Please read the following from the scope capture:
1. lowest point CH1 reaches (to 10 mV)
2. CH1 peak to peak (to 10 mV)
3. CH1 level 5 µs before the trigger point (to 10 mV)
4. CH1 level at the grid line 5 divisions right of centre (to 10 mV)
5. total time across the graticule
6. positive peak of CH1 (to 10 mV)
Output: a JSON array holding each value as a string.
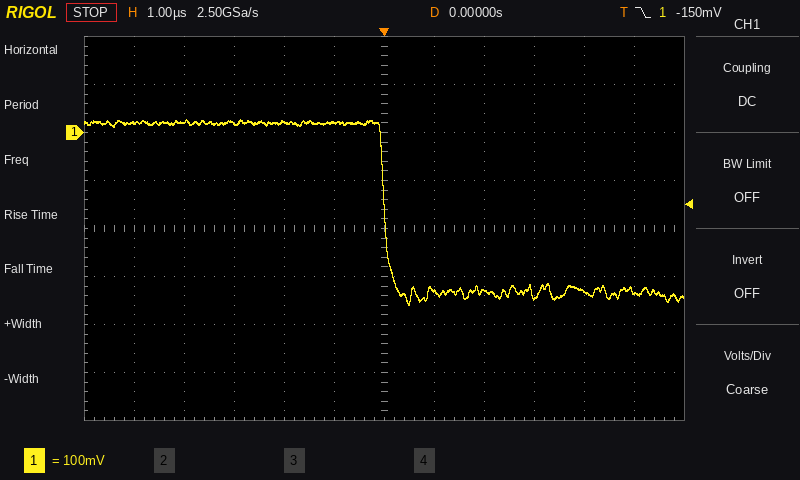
["-360 mV", "390 mV", "20 mV", "-330 mV", "12 µs", "30 mV"]
